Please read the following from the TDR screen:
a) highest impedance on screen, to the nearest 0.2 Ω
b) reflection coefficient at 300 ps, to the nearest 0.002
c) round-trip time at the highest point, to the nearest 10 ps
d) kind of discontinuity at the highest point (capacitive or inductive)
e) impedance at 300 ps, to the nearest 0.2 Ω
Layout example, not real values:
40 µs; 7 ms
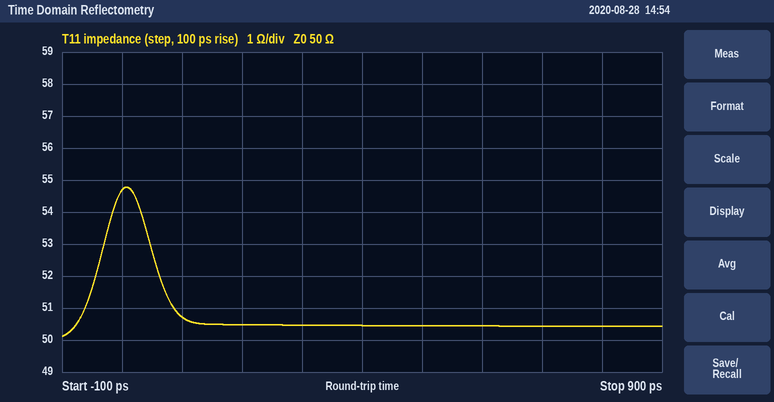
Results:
54.8 Ω; +0.004; 10 ps; inductive; 50.4 Ω
